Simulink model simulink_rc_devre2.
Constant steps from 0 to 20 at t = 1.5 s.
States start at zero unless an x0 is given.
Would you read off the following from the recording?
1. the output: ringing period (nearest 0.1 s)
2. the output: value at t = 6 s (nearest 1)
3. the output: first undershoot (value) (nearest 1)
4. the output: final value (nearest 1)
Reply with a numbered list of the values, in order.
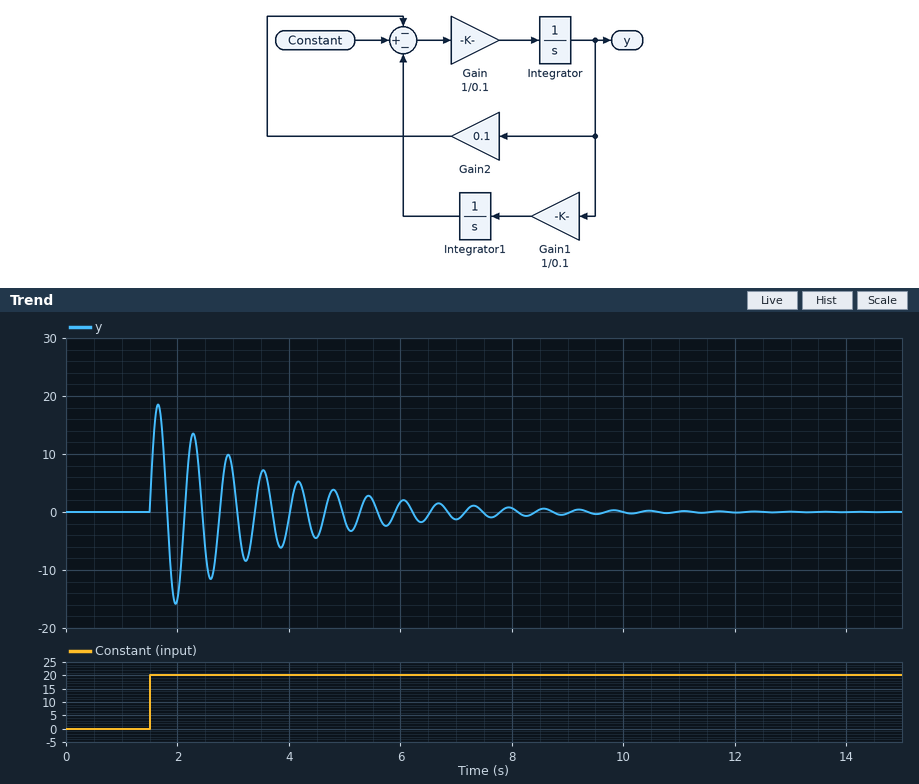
1. 0.6 s
2. 2
3. -16
4. 0
